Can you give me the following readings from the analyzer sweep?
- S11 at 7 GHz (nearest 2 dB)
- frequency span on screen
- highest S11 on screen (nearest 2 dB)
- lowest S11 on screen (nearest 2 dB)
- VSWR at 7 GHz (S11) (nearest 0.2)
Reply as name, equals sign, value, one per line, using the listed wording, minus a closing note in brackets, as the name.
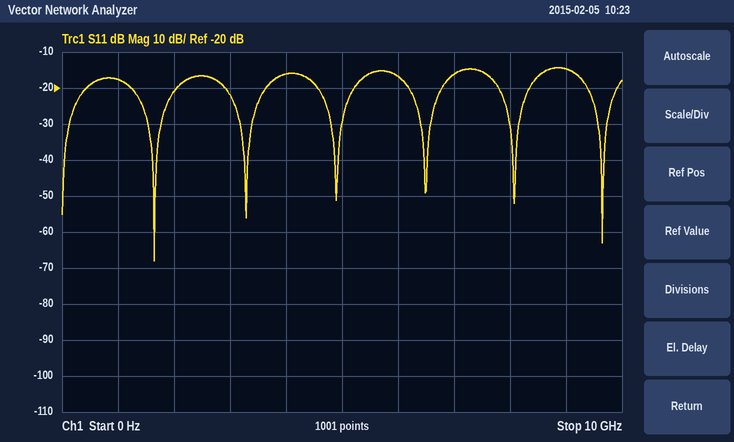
S11 at 7 GHz = -16 dB
frequency span on screen = 10 GHz
highest S11 on screen = -14 dB
lowest S11 on screen = -68 dB
VSWR at 7 GHz (S11) = 1.4
